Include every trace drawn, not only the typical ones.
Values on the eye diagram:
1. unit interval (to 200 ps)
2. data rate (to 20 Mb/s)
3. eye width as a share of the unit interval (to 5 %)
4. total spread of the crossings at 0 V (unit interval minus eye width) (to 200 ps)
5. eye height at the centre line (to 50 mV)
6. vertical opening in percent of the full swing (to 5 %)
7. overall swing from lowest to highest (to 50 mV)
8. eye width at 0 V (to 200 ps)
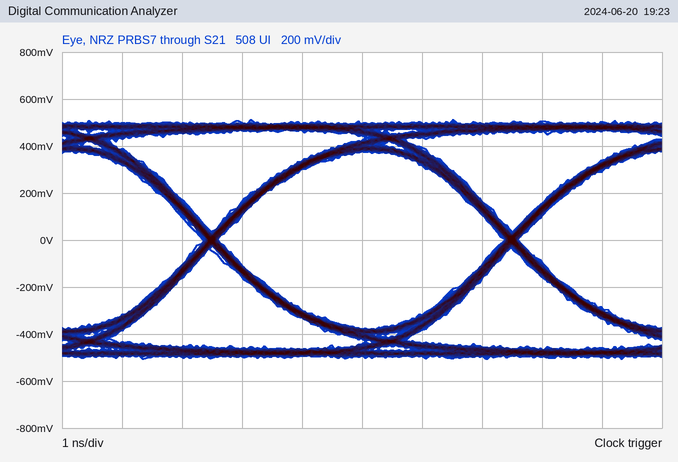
5.0 ns
200 Mb/s
95 %
200 ps
750 mV
75 %
1.00 V
4.8 ns
